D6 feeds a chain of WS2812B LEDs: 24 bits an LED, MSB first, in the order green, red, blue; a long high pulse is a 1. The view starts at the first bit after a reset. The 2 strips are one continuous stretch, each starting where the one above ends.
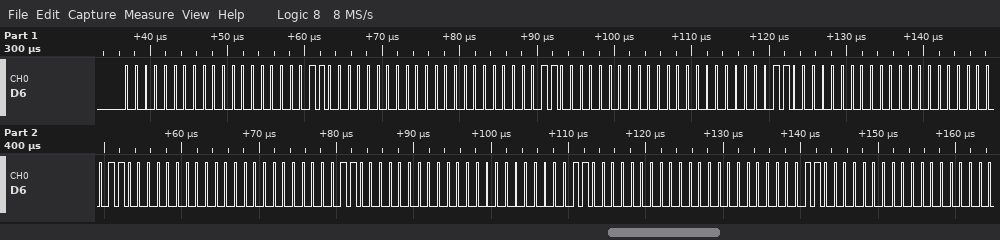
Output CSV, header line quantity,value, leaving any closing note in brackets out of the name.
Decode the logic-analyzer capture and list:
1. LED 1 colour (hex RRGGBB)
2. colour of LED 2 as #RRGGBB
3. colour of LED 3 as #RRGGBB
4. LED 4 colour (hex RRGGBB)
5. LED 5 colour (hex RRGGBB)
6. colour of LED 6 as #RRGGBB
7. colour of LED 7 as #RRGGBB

quantity,value
LED 1 colour,#000018
colour of LED 2 as #RRGGBB,#000018
colour of LED 3 as #RRGGBB,#000018
LED 4 colour,#000018
LED 5 colour,#000018
colour of LED 6 as #RRGGBB,#000018
colour of LED 7 as #RRGGBB,#000018
